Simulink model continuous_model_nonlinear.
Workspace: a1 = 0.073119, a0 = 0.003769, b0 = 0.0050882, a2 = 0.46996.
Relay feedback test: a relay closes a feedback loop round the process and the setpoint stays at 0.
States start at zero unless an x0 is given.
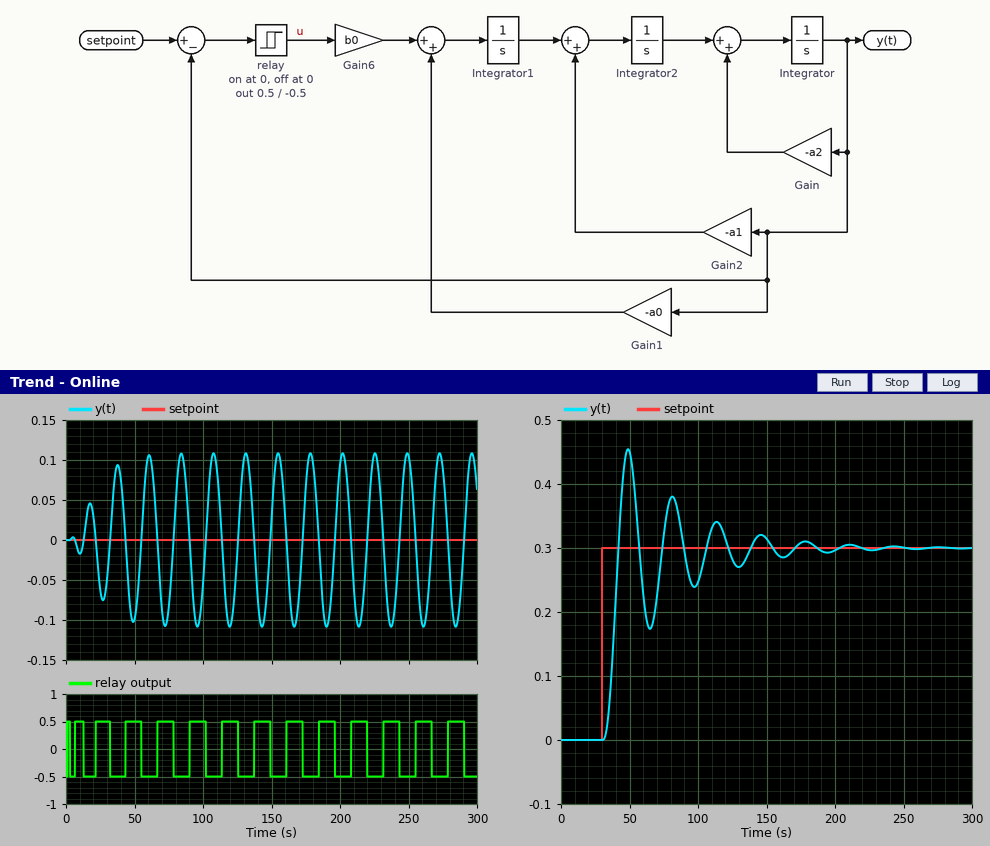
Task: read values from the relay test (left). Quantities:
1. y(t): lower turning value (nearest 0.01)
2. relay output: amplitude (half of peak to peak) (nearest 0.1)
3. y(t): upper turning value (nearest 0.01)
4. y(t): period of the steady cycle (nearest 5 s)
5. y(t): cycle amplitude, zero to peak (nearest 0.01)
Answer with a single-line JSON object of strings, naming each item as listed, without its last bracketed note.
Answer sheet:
{"y(t): lower turning value": "-0.11", "relay output: amplitude (half of peak to peak)": "0.5", "y(t): upper turning value": "0.11", "y(t): period of the steady cycle": "25 s", "y(t): cycle amplitude, zero to peak": "0.11"}
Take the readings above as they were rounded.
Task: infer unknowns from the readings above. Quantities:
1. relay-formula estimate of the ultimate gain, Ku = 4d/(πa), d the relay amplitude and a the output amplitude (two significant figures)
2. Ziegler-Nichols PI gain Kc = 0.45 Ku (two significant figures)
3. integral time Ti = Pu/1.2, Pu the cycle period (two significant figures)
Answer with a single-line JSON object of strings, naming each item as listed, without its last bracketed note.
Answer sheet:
{"relay-formula estimate of the ultimate gain, Ku = 4d/(πa), d the relay amplitude and a the output amplitude": "5.8", "Ziegler-Nichols PI gain Kc = 0.45 Ku": "2.6", "integral time Ti = Pu/1.2, Pu the cycle period": "21 s"}
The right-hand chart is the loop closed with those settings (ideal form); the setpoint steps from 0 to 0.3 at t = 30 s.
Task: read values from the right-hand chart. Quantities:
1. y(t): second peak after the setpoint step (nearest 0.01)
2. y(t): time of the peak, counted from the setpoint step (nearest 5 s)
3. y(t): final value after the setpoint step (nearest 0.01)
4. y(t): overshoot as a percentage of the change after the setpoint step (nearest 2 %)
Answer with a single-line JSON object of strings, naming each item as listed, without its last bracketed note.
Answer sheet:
{"y(t): second peak after the setpoint step": "0.38", "y(t): time of the peak, counted from the setpoint step": "20 s", "y(t): final value after the setpoint step": "0.30", "y(t): overshoot as a percentage of the change after the setpoint step": "52 %"}
